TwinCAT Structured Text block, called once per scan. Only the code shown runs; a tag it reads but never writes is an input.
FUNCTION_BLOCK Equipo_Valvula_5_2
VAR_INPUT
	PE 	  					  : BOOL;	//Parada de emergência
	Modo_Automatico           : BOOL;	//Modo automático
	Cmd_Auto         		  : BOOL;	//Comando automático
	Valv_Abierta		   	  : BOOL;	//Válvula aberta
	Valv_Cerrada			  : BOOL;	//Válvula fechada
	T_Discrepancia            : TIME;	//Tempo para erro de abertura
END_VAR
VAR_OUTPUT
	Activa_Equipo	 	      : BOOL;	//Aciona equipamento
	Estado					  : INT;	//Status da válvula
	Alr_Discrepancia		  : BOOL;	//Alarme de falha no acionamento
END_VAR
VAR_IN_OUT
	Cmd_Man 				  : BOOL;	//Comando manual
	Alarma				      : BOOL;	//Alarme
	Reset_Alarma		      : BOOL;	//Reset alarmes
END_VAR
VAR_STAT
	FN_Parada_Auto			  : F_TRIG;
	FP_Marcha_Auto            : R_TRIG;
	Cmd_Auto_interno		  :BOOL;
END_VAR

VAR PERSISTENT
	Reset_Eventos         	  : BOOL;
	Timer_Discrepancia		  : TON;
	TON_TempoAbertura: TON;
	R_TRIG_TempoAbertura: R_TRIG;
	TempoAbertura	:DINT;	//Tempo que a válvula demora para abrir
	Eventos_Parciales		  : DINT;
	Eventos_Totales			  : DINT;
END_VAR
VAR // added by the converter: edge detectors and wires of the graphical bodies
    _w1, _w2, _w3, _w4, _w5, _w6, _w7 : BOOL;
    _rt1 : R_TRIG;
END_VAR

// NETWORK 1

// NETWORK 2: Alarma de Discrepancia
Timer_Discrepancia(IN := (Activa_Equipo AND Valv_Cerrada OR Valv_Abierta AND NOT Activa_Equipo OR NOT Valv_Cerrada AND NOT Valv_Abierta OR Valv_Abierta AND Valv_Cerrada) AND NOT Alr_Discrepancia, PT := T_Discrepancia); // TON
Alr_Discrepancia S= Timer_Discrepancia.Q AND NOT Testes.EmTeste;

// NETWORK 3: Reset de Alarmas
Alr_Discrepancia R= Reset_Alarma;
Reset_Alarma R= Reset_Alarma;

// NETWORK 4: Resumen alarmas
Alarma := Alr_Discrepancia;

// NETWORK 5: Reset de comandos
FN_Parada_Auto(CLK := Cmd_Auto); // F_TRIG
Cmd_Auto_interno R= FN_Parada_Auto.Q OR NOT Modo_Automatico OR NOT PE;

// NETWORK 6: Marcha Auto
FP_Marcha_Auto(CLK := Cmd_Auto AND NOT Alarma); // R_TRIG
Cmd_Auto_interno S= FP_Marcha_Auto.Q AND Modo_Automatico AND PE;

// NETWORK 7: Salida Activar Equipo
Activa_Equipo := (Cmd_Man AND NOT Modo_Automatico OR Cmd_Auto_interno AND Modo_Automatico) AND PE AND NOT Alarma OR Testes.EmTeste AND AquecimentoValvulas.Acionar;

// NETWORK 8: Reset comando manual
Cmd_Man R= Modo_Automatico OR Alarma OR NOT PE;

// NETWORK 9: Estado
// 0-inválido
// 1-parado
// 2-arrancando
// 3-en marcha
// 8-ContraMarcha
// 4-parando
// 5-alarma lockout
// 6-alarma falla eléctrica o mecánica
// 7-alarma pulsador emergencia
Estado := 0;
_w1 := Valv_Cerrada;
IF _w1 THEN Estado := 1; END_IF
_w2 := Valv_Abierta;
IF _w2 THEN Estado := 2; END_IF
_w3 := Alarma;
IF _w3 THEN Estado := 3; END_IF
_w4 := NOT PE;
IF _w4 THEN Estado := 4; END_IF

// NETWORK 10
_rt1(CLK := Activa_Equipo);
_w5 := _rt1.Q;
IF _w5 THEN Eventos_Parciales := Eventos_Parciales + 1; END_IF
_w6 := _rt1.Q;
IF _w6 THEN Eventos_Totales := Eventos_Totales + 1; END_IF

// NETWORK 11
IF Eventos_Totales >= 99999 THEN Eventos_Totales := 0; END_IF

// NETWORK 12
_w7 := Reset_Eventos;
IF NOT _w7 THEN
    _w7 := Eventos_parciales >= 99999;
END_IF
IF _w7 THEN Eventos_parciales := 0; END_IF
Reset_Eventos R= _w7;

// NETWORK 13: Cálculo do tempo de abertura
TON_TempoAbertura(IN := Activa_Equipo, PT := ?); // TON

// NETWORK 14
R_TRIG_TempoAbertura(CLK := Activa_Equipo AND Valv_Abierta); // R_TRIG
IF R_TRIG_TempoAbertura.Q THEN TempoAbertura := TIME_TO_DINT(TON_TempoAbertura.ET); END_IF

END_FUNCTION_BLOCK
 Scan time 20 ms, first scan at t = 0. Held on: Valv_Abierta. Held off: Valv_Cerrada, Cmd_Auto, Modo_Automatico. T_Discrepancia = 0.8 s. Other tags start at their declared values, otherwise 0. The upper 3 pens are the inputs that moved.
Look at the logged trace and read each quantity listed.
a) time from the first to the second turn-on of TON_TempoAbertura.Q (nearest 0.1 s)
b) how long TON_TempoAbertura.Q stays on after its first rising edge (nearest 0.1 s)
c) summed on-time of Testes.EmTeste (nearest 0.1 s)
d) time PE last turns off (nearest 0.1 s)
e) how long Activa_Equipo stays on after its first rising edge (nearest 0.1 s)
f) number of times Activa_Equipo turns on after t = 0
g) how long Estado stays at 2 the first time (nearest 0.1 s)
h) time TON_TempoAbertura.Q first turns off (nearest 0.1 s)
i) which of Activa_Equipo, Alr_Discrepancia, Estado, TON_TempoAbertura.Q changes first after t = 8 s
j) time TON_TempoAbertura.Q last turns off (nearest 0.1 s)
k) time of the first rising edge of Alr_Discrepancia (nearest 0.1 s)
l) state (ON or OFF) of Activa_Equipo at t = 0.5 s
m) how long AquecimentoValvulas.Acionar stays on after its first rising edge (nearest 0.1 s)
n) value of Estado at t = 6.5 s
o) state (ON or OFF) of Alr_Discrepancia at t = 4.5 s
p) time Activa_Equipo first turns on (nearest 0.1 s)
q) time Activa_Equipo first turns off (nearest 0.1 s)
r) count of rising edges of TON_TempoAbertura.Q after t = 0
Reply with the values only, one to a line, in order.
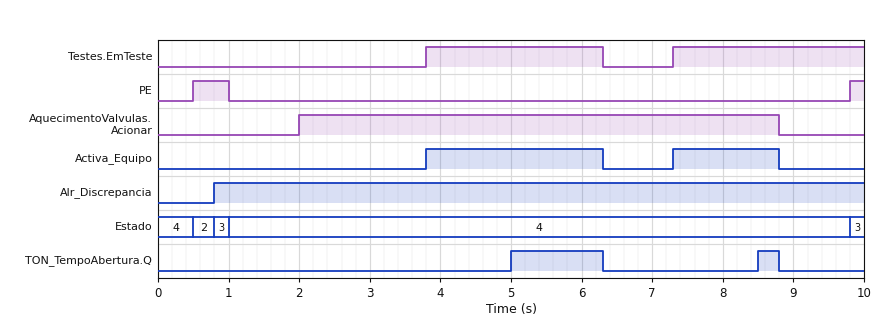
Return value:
3.5 s
1.3 s
5.2 s
1.0 s
2.5 s
2
0.3 s
6.3 s
TON_TempoAbertura.Q
8.8 s
0.8 s
OFF
6.8 s
4
ON
3.8 s
6.3 s
2
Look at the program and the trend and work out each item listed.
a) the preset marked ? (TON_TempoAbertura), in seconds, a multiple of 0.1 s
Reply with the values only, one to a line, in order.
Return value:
1.2 s
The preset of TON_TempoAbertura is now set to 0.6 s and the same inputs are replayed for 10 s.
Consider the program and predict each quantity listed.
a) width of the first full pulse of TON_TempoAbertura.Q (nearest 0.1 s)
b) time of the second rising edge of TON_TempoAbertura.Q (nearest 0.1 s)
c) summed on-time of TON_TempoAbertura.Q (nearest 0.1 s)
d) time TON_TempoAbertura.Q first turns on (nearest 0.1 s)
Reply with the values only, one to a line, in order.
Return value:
1.9 s
7.9 s
2.8 s
4.4 s
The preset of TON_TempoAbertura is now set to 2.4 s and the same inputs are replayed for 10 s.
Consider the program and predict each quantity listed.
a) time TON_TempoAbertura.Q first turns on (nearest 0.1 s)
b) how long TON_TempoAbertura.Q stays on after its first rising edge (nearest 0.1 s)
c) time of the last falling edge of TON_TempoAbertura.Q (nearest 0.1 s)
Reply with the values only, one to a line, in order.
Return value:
6.2 s
0.1 s
6.3 s
